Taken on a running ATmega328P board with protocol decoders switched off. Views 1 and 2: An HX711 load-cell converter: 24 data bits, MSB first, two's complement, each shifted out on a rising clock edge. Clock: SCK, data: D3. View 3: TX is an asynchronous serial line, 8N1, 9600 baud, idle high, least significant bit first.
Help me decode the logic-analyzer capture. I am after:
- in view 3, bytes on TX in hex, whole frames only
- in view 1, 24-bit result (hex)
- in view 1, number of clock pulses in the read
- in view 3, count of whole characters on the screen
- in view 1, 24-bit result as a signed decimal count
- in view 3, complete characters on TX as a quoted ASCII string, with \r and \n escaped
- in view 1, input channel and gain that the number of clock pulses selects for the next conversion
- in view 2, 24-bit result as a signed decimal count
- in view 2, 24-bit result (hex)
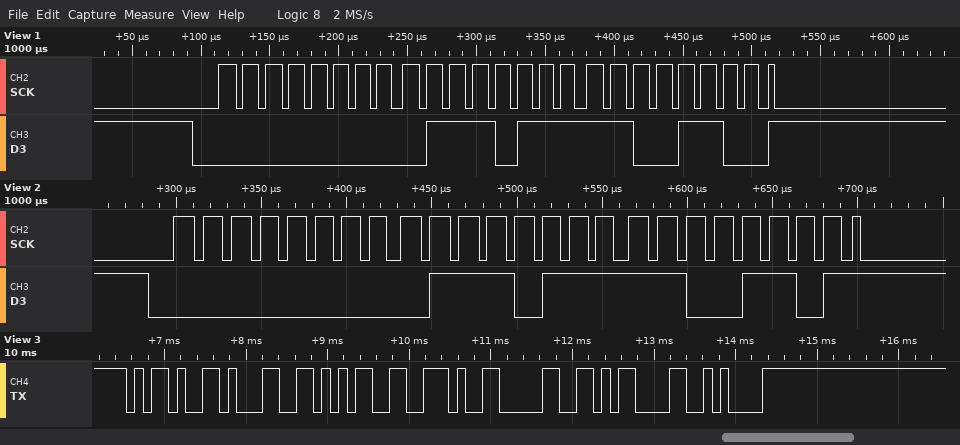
2D 31 35 2E 30 0D 0A
0x0077CC
25
7
30668
"-15.0\r\n"
channel A, gain 128
30669
0x0077CD
